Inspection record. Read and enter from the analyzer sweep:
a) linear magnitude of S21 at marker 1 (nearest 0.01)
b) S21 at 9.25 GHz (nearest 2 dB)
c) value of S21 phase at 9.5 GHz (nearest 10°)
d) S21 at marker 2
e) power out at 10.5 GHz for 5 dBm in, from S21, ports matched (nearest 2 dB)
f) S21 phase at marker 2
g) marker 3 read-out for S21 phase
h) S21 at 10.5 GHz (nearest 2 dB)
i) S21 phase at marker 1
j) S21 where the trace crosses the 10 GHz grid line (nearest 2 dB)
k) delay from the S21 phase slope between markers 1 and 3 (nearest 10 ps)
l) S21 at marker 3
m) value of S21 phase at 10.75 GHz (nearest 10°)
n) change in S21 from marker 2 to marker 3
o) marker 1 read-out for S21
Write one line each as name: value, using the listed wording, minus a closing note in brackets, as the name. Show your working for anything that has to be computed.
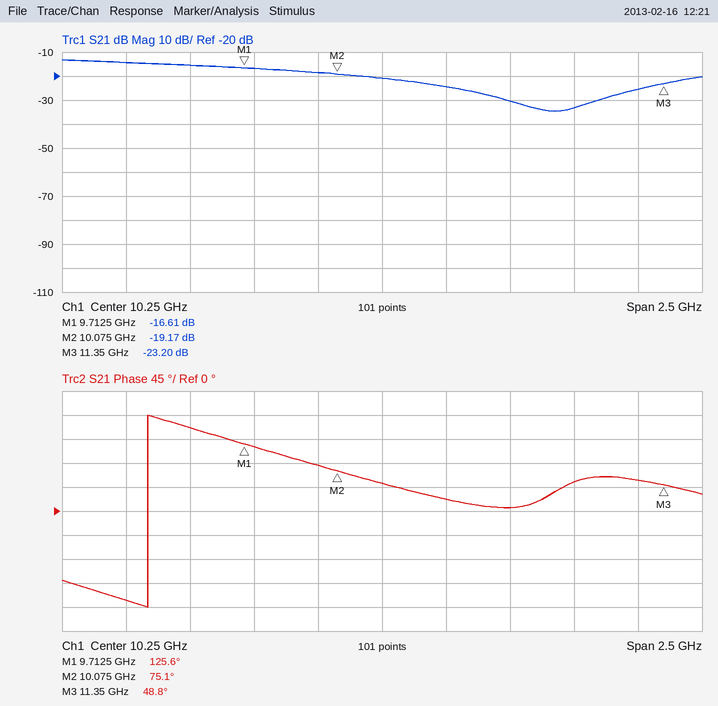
linear magnitude of S21 at marker 1: 10^(-16.61/20) ≈ 0.15
S21 at 9.25 GHz: -14 dB
value of S21 phase at 9.5 GHz: 160°
S21 at marker 2: -19.17 dB
power out at 10.5 GHz for 5 dBm in, from S21, ports matched: 5 dBm + (-24 dB) = -20 dBm
S21 phase at marker 2: 75.1°
marker 3 read-out for S21 phase: 48.8°
S21 at 10.5 GHz: -24 dB
S21 phase at marker 1: 125.6°
S21 where the trace crosses the 10 GHz grid line: -18 dB
delay from the S21 phase slope between markers 1 and 3: −(48.8° − (125.6°))/(360° × 1.6375 GHz) ≈ 130 ps
S21 at marker 3: -23.20 dB
value of S21 phase at 10.75 GHz: 10°
change in S21 from marker 2 to marker 3: -23.2 − (-19.17) = -4.03 dB
marker 1 read-out for S21: -16.61 dB
